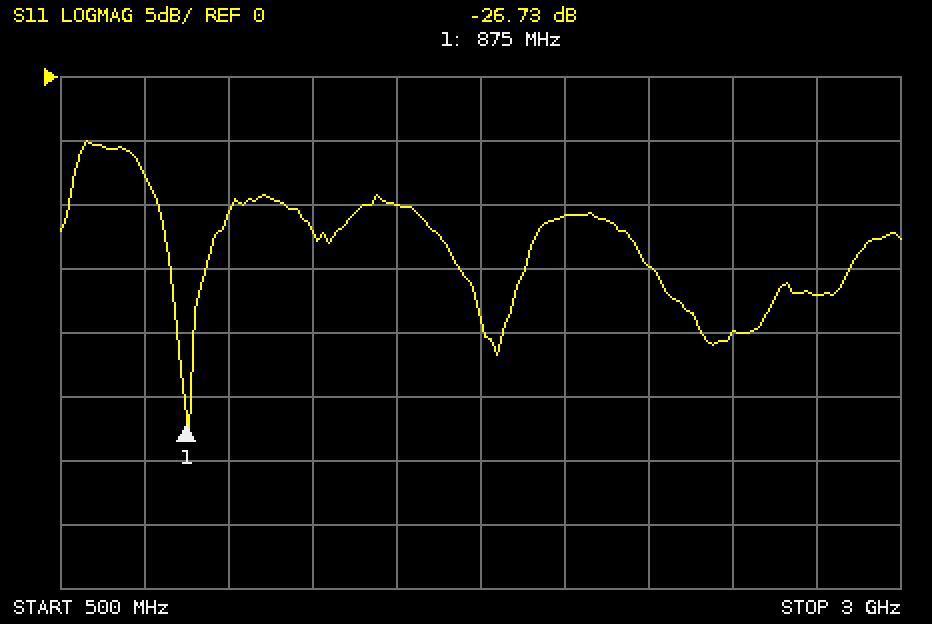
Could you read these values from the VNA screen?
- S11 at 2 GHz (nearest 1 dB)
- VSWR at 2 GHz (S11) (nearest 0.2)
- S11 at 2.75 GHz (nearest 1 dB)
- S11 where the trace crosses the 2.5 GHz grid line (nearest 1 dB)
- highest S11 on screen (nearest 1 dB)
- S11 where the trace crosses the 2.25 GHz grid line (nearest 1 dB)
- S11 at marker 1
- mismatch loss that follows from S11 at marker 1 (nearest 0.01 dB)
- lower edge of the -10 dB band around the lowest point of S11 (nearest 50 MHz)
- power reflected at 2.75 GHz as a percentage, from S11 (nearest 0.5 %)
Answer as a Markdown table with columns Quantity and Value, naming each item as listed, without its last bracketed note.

| Quantity | Value |
|---|---|
| S11 at 2 GHz | -11 dB |
| VSWR at 2 GHz (S11) | 1.8 |
| S11 at 2.75 GHz | -17 dB |
| S11 where the trace crosses the 2.5 GHz grid line | -20 dB |
| highest S11 on screen | -5 dB |
| S11 where the trace crosses the 2.25 GHz grid line | -15 dB |
| S11 at marker 1 | -26.73 dB |
| mismatch loss that follows from S11 at marker 1 | 0.01 dB |
| lower edge of the -10 dB band around the lowest point of S11 | 800 MHz |
| power reflected at 2.75 GHz as a percentage, from S11 | 2.0 % |
